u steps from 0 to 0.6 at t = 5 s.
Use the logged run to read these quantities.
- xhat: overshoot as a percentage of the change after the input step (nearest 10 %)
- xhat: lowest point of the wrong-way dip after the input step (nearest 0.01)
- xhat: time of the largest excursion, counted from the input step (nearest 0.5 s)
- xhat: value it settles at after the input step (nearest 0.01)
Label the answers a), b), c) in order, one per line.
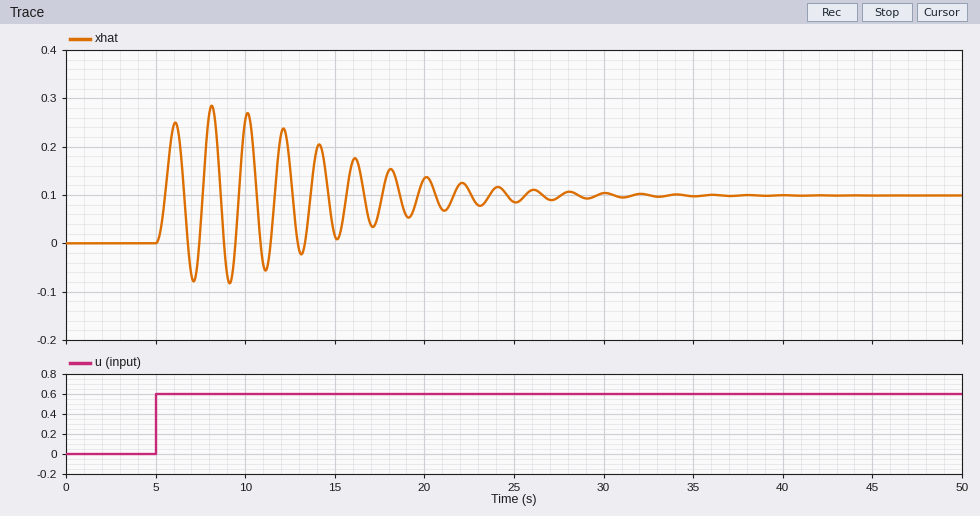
a) 190 %
b) -0.08
c) 3.0 s
d) 0.10
